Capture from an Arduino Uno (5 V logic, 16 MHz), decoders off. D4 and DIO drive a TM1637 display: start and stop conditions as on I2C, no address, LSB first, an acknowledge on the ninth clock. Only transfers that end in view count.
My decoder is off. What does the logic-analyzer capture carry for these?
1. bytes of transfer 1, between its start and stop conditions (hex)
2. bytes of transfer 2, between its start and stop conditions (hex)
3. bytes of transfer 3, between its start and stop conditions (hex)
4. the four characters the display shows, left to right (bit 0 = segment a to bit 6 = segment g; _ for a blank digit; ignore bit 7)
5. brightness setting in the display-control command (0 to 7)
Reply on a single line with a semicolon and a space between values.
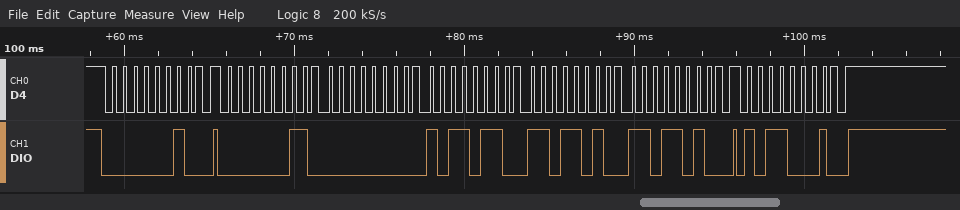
40; C0 00 6D 5B 5B; 8D; _522; 5
